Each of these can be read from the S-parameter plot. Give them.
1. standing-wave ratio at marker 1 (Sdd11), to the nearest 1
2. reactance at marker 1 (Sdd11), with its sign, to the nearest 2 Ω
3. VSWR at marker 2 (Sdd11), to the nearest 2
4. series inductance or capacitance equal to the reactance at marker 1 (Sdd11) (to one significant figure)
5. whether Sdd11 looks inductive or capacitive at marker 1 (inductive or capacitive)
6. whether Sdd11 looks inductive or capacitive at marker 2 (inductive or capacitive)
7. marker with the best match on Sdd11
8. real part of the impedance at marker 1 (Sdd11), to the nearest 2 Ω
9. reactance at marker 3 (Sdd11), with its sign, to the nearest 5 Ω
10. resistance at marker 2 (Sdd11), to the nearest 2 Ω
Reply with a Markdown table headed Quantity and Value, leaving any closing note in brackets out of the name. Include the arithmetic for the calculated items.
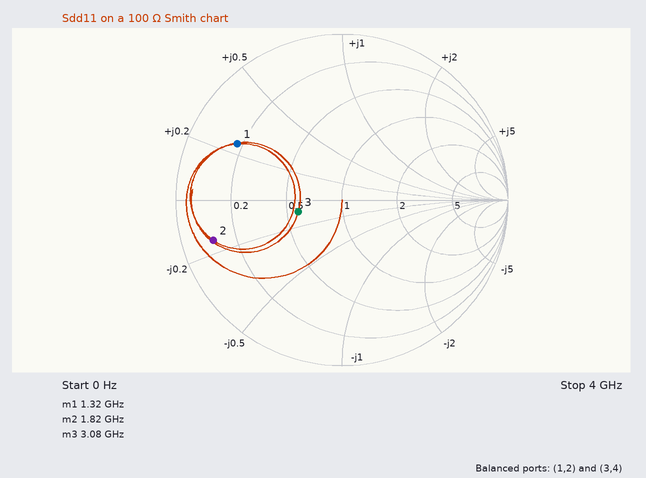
| Quantity | Value |
|---|---|
| standing-wave ratio at marker 1 (Sdd11), to the nearest 1 | 6 |
| reactance at marker 1 (Sdd11), with its sign, to the nearest 2 Ω | +24 Ω |
| VSWR at marker 2 (Sdd11), to the nearest 2 | 10 |
| series inductance or capacitance equal to the reactance at marker 1 (Sdd11) | L = 24 Ω/(2π × 1.32 GHz) ≈ 3 nH |
| whether Sdd11 looks inductive or capacitive at marker 1 | inductive |
| whether Sdd11 looks inductive or capacitive at marker 2 | capacitive |
| marker with the best match on Sdd11 | marker 3 |
| real part of the impedance at marker 1 (Sdd11), to the nearest 2 Ω | 18 Ω |
| reactance at marker 3 (Sdd11), with its sign, to the nearest 5 Ω | -10 Ω |
| resistance at marker 2 (Sdd11), to the nearest 2 Ω | 10 Ω |
